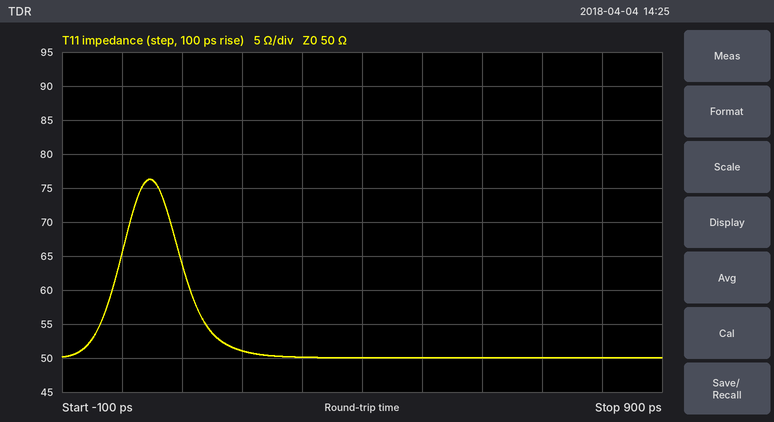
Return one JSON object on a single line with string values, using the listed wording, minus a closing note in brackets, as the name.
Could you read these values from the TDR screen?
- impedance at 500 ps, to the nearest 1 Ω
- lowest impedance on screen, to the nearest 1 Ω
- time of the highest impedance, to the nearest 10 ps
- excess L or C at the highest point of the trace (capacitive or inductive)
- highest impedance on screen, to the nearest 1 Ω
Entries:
{"impedance at 500 ps, to the nearest 1 Ω": "50 Ω", "lowest impedance on screen, to the nearest 1 Ω": "50 Ω", "time of the highest impedance, to the nearest 10 ps": "50 ps", "excess L or C at the highest point of the trace": "inductive", "highest impedance on screen, to the nearest 1 Ω": "76 Ω"}
